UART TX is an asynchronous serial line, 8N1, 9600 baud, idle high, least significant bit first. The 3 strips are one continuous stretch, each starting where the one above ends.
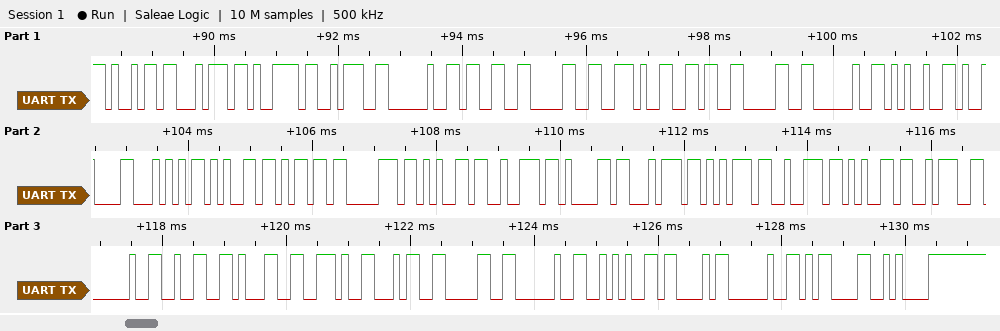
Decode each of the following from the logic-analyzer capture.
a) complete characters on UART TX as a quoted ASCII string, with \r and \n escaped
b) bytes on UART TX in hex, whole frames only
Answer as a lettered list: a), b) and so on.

a) "ity: 30.60 %\tTemperature: 21.40 *C \r\n"
b) 69 74 79 3A 20 33 30 2E 36 30 20 25 09 54 65 6D 70 65 72 61 74 75 72 65 3A 20 32 31 2E 34 30 20 2A 43 20 0D 0A
